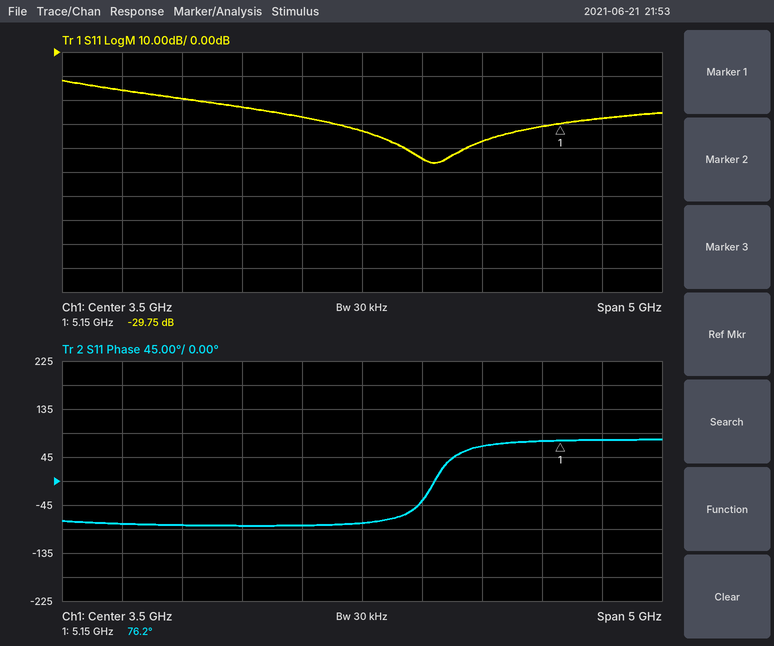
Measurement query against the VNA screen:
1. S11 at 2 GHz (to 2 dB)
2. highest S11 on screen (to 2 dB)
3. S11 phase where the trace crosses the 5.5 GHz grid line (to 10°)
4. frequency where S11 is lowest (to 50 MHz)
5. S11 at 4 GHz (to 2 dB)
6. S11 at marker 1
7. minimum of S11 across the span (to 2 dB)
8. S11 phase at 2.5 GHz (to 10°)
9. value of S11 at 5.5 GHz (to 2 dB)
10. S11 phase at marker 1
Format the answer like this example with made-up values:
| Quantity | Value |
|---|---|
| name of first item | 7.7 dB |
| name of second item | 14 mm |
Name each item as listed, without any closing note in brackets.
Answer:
| Quantity | Value |
|---|---|
| S11 at 2 GHz | -20 dB |
| highest S11 on screen | -12 dB |
| S11 phase where the trace crosses the 5.5 GHz grid line | 80° |
| frequency where S11 is lowest | 4.10 GHz |
| S11 at 4 GHz | -44 dB |
| S11 at marker 1 | -29.75 dB |
| minimum of S11 across the span | -46 dB |
| S11 phase at 2.5 GHz | -80° |
| value of S11 at 5.5 GHz | -28 dB |
| S11 phase at marker 1 | 76.2° |
